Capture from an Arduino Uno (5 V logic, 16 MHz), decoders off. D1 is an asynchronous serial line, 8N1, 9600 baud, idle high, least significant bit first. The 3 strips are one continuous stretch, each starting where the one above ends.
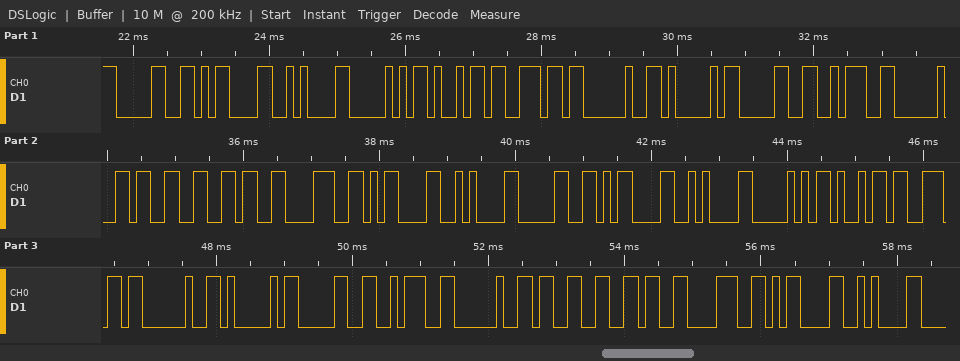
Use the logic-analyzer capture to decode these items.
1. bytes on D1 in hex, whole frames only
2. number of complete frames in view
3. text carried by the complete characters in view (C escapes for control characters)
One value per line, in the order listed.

30 0D 0A 50 69 6E 20 41 30 3A 20 33 36 38 0D 0A 30 0D 0A 50 69 6E 20 41 30 3A 20 33 36 38 0D 0A
32
"0\r\nPin A0: 368\r\n0\r\nPin A0: 368\r\n"
